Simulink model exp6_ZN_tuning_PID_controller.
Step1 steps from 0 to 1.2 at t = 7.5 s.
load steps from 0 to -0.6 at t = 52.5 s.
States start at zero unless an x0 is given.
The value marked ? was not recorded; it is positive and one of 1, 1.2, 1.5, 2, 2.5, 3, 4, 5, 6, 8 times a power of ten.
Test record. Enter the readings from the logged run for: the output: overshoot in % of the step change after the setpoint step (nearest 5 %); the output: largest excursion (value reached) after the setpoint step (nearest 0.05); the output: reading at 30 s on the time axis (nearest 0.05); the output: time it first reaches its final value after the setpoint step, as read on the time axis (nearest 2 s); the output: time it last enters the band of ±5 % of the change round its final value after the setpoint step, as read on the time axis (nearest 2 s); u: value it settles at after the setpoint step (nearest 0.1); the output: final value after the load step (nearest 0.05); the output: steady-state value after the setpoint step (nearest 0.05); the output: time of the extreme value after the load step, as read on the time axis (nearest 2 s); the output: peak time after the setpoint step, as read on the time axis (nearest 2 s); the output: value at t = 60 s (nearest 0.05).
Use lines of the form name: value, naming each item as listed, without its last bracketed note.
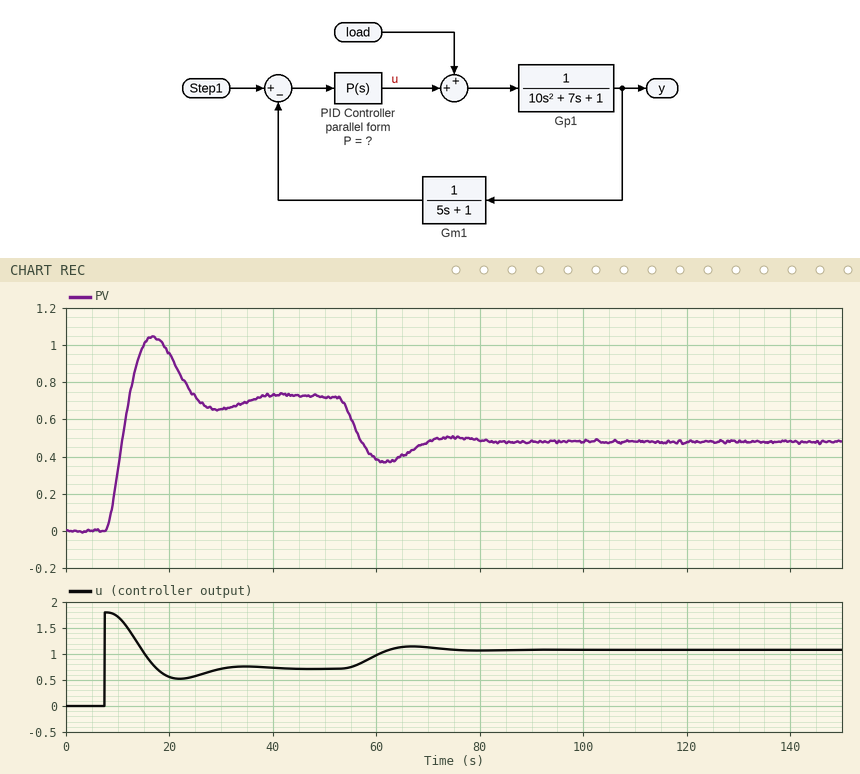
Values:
the output: overshoot in % of the step change after the setpoint step: 45 %
the output: largest excursion (value reached) after the setpoint step: 1.05
the output: reading at 30 s on the time axis: 0.65
the output: time it first reaches its final value after the setpoint step, as read on the time axis: 12 s
the output: time it last enters the band of ±5 % of the change round its final value after the setpoint step, as read on the time axis: 34 s
u: value it settles at after the setpoint step: 0.7
the output: final value after the load step: 0.50
the output: steady-state value after the setpoint step: 0.70
the output: time of the extreme value after the load step, as read on the time axis: 62 s
the output: peak time after the setpoint step, as read on the time axis: 16 s
the output: value at t = 60 s: 0.40
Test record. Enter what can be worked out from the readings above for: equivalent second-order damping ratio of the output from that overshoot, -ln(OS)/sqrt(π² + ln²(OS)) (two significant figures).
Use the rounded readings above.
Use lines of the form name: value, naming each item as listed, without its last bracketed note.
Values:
equivalent second-order damping ratio of the output from that overshoot, -ln(OS)/sqrt(π² + ln²(OS)): 0.25
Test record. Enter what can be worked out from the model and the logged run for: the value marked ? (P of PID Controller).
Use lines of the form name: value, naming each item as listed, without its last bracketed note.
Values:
the value marked ?: 1.5
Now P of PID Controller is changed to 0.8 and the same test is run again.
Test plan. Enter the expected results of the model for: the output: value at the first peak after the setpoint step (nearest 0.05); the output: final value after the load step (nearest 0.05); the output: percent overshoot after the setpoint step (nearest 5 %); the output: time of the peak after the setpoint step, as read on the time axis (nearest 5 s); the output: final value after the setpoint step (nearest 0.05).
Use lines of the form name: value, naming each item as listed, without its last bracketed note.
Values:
the output: value at the first peak after the setpoint step: 0.65
the output: final value after the load step: 0.20
the output: percent overshoot after the setpoint step: 20 %
the output: time of the peak after the setpoint step, as read on the time axis: 20 s
the output: final value after the setpoint step: 0.55
